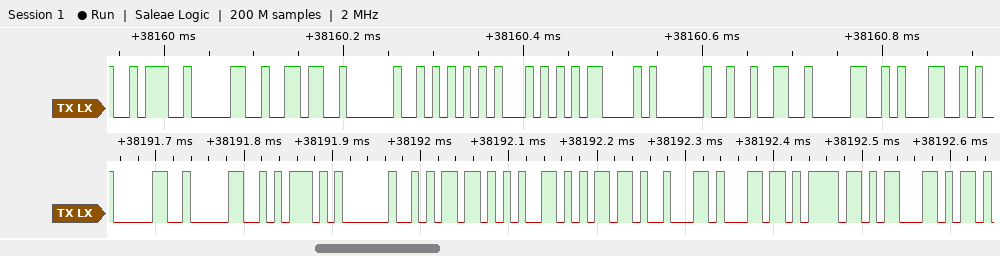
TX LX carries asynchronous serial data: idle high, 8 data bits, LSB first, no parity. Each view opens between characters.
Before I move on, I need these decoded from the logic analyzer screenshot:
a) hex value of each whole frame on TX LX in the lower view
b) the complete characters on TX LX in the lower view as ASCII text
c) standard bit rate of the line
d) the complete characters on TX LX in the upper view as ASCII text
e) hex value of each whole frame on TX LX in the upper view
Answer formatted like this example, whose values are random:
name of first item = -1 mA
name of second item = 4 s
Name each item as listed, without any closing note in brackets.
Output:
hex value of each whole frame on TX LX in the lower view = 30, 30, 5D, 20, 6D, 65, 6D, 62, 6C, 6F, 63
the complete characters on TX LX in the lower view as ASCII text = "00] membloc"
standard bit rate of the line = 115200 baud
the complete characters on TX LX in the upper view as ASCII text = ":06 UTC 201"
hex value of each whole frame on TX LX in the upper view = 3A, 30, 36, 20, 55, 54, 43, 20, 32, 30, 31
